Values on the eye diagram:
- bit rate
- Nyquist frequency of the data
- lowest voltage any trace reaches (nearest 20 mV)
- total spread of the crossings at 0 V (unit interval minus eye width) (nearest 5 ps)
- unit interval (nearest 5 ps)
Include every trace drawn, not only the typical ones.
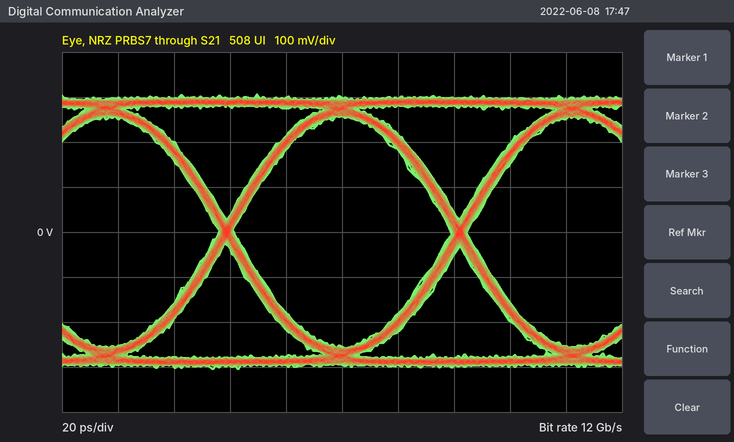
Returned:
12 Gb/s
6 GHz
-300 mV
5 ps
85 ps
